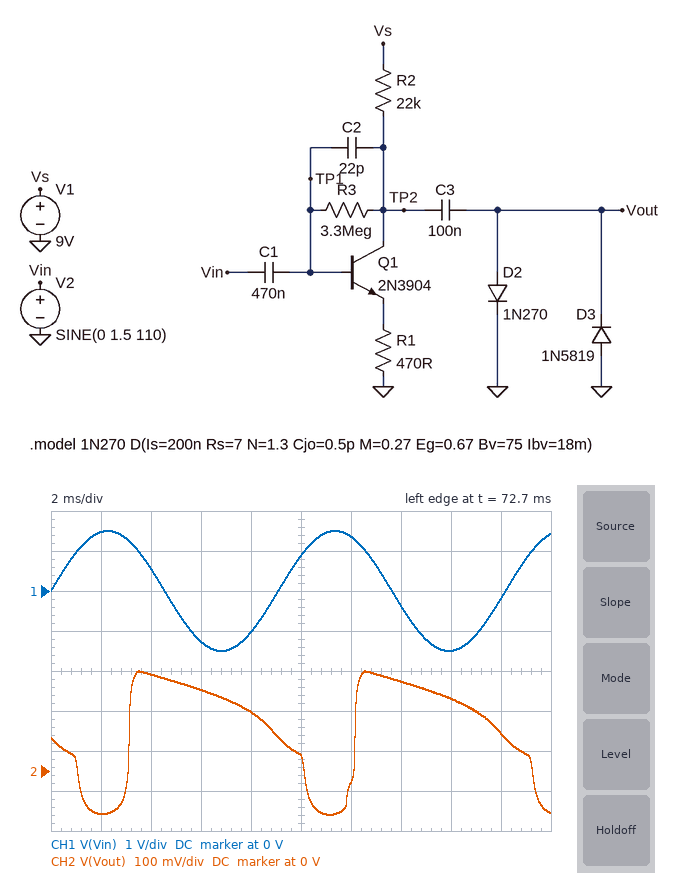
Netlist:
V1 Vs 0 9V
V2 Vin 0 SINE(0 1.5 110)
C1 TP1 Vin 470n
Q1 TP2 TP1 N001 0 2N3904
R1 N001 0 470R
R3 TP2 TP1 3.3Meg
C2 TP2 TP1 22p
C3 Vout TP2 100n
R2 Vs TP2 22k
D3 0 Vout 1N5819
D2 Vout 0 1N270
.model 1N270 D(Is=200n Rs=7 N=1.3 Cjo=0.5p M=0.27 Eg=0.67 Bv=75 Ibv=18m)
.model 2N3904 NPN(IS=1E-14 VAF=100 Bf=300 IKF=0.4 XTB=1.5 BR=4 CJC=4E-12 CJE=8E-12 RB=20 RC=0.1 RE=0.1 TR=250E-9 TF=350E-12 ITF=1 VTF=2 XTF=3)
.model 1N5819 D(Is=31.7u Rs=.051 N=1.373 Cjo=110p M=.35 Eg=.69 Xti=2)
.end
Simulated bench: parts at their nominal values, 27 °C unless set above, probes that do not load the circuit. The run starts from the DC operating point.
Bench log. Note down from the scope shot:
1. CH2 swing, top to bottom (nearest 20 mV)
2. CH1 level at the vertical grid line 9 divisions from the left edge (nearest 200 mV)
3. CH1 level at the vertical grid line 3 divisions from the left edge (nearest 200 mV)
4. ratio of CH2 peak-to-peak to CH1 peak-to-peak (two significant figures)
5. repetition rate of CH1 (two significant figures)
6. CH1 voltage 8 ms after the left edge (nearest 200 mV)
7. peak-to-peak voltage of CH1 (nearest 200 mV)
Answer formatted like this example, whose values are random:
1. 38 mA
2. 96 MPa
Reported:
1. 360 mV
2. -200 mV
3. -1.2 V
4. 0.12
5. 110 Hz
6. -1.0 V
7. 3.0 V
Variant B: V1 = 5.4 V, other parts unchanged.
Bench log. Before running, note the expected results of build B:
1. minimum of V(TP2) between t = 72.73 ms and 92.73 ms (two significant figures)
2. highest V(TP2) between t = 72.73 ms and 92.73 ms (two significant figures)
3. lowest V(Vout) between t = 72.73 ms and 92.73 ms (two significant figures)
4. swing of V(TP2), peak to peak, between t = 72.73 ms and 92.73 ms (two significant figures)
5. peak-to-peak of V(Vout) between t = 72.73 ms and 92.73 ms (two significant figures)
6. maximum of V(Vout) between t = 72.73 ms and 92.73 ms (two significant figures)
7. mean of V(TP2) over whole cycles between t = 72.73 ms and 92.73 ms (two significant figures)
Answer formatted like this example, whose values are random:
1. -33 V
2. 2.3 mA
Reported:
1. 170 mV
2. 5.1 V
3. -98 mV
4. 4.9 V
5. 330 mV
6. 230 mV
7. 3.6 V
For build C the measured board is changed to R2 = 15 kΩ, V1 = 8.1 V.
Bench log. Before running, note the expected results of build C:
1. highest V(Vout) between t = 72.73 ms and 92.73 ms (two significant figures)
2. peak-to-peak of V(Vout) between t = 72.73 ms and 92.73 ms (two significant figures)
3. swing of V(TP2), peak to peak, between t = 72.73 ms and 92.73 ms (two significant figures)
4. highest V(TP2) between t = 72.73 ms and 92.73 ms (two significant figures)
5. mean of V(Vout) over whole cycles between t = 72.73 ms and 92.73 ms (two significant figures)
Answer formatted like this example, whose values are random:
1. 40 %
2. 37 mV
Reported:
1. 260 mV
2. 360 mV
3. 7.6 V
4. 7.9 V
5. 90 mV
